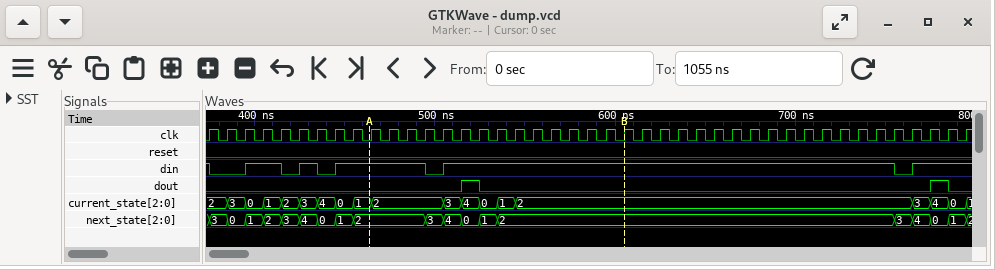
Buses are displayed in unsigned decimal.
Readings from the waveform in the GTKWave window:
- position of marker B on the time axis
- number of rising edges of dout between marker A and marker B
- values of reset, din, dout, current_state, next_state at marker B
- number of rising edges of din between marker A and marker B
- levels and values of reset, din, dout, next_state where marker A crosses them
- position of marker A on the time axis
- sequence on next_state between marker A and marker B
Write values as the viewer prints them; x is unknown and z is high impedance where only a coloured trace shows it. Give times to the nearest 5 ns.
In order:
605 ns
1
reset=0, din=1, dout=0, current_state=2, next_state=2
1
reset=0, din=1, dout=0, next_state=2
465 ns
2, 3, 4, 0, 1, 2
